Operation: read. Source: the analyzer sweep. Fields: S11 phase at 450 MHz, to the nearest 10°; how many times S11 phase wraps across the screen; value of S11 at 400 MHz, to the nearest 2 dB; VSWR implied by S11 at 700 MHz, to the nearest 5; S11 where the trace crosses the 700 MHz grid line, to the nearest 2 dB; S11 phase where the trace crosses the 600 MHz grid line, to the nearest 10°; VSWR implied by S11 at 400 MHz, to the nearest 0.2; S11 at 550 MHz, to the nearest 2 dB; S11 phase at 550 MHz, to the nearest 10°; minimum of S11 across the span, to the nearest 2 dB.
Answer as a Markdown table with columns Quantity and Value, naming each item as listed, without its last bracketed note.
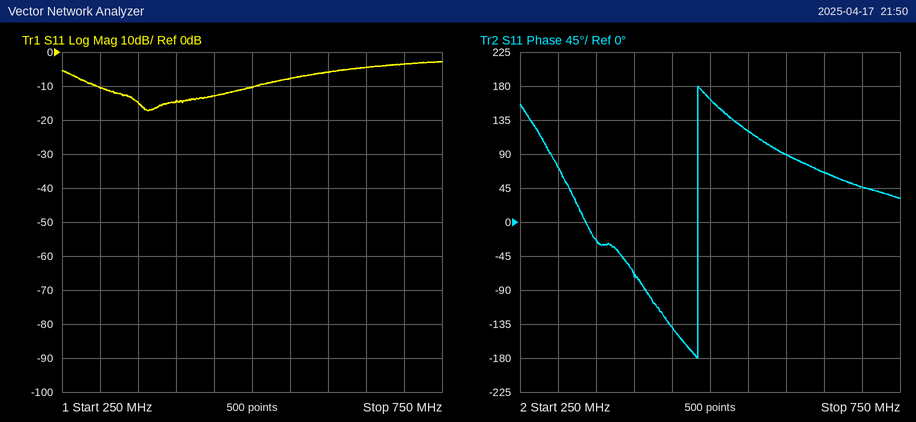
| Quantity | Value |
|---|---|
| S11 phase at 450 MHz, to the nearest 10° | -140° |
| how many times S11 phase wraps across the screen | 1 |
| value of S11 at 400 MHz, to the nearest 2 dB | -14 dB |
| VSWR implied by S11 at 700 MHz, to the nearest 5 | 5 |
| S11 where the trace crosses the 700 MHz grid line, to the nearest 2 dB | -4 dB |
| S11 phase where the trace crosses the 600 MHz grid line, to the nearest 10° | 90° |
| VSWR implied by S11 at 400 MHz, to the nearest 0.2 | 1.4 |
| S11 at 550 MHz, to the nearest 2 dB | -8 dB |
| S11 phase at 550 MHz, to the nearest 10° | 120° |
| minimum of S11 across the span, to the nearest 2 dB | -18 dB |
